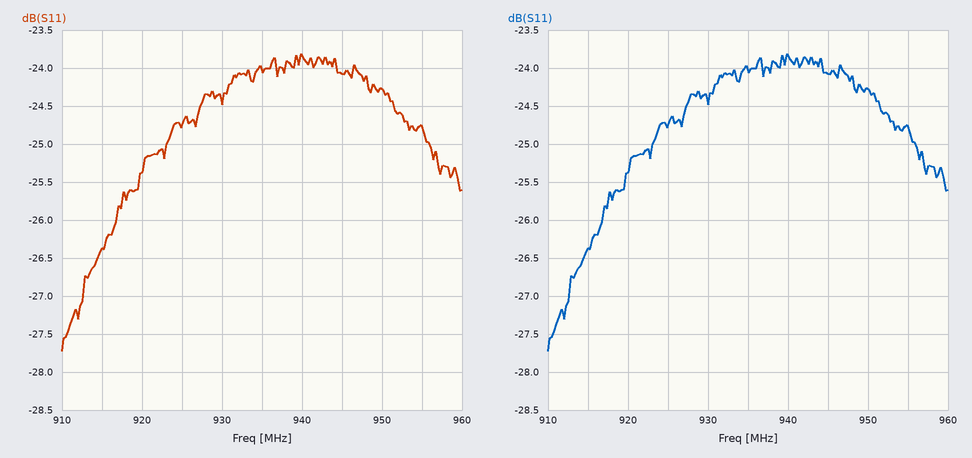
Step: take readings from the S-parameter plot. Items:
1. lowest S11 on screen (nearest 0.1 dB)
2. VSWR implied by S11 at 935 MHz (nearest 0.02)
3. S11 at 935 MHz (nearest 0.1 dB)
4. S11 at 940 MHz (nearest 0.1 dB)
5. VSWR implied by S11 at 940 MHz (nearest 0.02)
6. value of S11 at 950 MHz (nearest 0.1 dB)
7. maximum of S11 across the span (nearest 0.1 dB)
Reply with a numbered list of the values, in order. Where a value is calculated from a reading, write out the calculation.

1. -27.7 dB
2. |Γ| = 10^(-24/20) = 0.0631; VSWR = (1 + 0.0631)/(1 − 0.0631) ≈ 1.13, so 1.14 to the nearest 0.02
3. -24.0 dB
4. -23.8 dB
5. |Γ| = 10^(-23.8/20) = 0.0646; VSWR = (1 + 0.0646)/(1 − 0.0646) ≈ 1.14
6. -24.3 dB
7. -23.8 dB
